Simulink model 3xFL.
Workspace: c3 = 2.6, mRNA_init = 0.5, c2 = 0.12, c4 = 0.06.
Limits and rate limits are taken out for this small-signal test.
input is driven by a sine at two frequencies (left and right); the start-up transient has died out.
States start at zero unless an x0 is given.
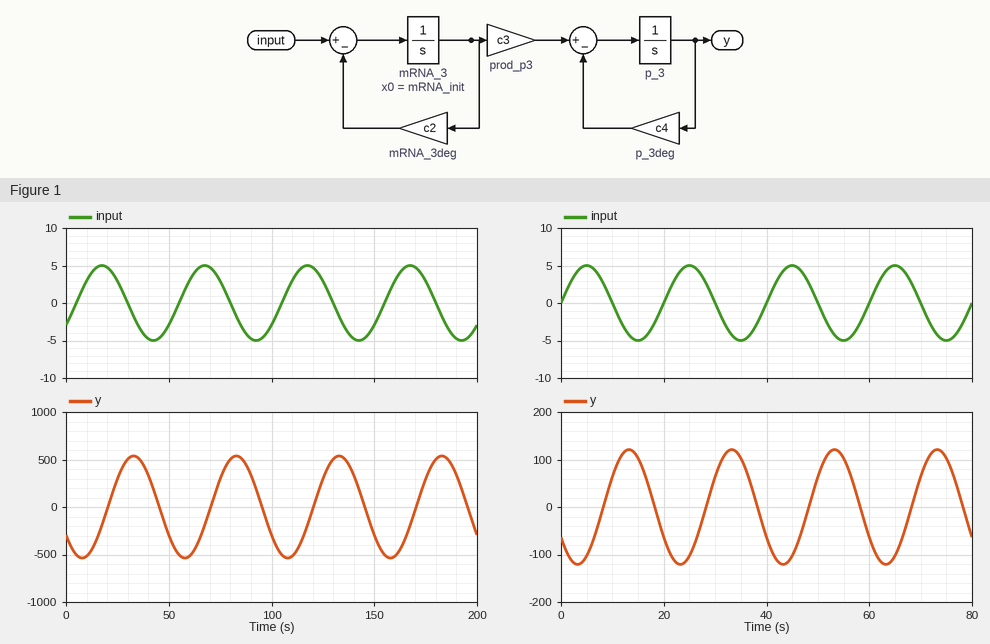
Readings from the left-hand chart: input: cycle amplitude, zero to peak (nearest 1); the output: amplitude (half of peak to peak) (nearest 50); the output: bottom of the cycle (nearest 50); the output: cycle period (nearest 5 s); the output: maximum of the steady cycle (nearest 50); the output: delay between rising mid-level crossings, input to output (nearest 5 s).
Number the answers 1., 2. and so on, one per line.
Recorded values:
1. 5
2. 550
3. -550
4. 50 s
5. 550
6. 15 s
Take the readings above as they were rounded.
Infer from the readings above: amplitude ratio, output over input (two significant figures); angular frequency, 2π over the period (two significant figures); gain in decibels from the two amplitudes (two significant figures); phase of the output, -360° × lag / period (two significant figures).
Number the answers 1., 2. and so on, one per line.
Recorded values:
1. 110
2. 0.13 rad/s
3. 41 dB
4. -110°
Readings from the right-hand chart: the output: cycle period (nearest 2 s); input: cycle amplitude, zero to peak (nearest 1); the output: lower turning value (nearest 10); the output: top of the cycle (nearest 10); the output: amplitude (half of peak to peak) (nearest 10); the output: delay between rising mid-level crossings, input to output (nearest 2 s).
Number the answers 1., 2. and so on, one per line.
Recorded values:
1. 20 s
2. 5
3. -120
4. 120
5. 120
6. 8 s
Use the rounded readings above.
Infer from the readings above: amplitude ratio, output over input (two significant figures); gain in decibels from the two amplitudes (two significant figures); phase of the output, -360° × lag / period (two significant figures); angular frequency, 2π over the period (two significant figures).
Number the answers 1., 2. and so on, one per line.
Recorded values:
1. 24
2. 28 dB
3. -140°
4. 0.31 rad/s
